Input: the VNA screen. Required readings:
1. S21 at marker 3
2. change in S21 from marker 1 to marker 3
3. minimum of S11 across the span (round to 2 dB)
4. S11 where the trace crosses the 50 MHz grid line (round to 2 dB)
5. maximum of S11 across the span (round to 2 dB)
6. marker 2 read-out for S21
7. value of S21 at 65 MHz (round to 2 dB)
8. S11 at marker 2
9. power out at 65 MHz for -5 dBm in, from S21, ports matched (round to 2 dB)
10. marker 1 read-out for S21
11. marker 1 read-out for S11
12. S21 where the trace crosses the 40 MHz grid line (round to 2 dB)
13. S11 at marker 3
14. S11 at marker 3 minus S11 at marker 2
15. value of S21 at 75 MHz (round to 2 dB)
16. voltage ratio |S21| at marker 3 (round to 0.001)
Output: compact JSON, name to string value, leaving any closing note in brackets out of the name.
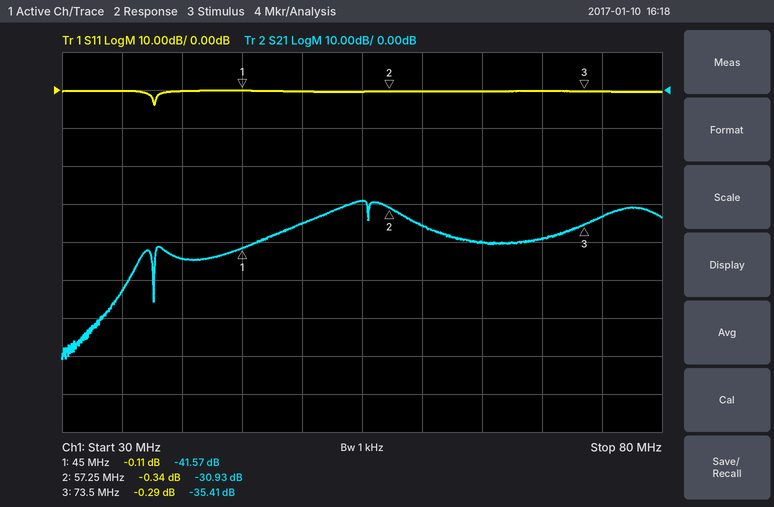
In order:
{"S21 at marker 3": "-35.41 dB", "change in S21 from marker 1 to marker 3": "6.16 dB", "minimum of S11 across the span": "-4 dB", "S11 where the trace crosses the 50 MHz grid line": "0 dB", "maximum of S11 across the span": "0 dB", "marker 2 read-out for S21": "-30.93 dB", "value of S21 at 65 MHz": "-40 dB", "S11 at marker 2": "-0.34 dB", "power out at 65 MHz for -5 dBm in, from S21, ports matched": "-46 dBm", "marker 1 read-out for S21": "-41.57 dB", "marker 1 read-out for S11": "-0.11 dB", "S21 where the trace crosses the 40 MHz grid line": "-44 dB", "S11 at marker 3": "-0.29 dB", "S11 at marker 3 minus S11 at marker 2": "0.05 dB", "value of S21 at 75 MHz": "-34 dB", "voltage ratio |S21| at marker 3": "0.017"}
